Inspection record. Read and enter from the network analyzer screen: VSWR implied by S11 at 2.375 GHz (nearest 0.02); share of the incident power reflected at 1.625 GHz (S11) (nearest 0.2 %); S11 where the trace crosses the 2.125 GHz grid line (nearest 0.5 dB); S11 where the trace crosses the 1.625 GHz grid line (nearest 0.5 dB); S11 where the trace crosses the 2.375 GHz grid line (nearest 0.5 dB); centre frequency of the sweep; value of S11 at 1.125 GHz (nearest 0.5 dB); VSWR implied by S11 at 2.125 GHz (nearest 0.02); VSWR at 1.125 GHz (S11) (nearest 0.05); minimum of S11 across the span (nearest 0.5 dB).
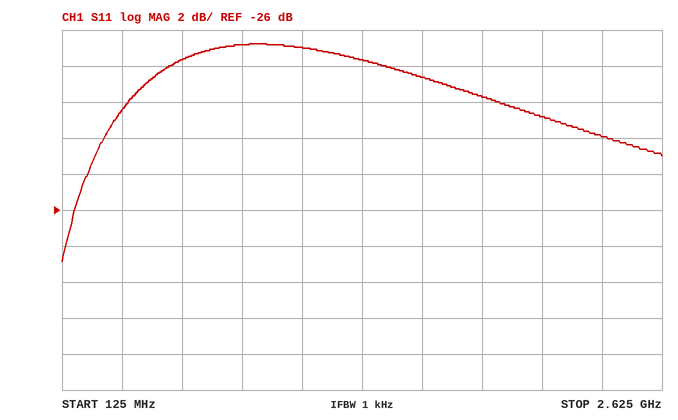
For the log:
1.18
1.4 %
-21.0 dB
-18.5 dB
-22.0 dB
1.375 GHz
-17.0 dB
1.20
1.35
-29.0 dB
